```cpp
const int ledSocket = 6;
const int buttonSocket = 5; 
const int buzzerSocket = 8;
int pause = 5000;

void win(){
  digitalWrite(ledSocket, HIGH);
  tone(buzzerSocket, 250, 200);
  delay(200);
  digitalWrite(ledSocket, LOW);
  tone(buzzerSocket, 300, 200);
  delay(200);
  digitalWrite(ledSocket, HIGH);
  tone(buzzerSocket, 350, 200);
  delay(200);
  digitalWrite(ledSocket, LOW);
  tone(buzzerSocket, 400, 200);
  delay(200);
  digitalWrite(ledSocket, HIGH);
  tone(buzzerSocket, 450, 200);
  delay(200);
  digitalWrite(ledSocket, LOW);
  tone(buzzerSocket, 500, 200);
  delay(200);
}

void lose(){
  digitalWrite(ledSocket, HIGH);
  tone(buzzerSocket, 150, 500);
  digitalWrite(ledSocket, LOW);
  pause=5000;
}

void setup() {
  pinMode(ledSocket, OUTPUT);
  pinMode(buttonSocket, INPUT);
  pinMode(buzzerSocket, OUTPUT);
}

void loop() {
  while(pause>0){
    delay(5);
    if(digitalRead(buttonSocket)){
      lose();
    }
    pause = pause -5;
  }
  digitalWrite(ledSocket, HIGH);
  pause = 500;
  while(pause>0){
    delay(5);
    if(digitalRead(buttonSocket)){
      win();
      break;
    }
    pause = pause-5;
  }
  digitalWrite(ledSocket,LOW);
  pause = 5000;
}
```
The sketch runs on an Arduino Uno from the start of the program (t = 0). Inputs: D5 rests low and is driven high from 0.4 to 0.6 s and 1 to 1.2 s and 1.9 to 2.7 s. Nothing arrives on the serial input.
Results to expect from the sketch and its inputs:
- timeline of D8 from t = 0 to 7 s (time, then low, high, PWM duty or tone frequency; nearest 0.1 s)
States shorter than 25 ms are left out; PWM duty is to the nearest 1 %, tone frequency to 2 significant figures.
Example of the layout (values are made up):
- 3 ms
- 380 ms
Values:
- 0 s low; 0.4 s tone 150 Hz; 1.7 s low; 1.9 s tone 150 Hz; 3.2 s low
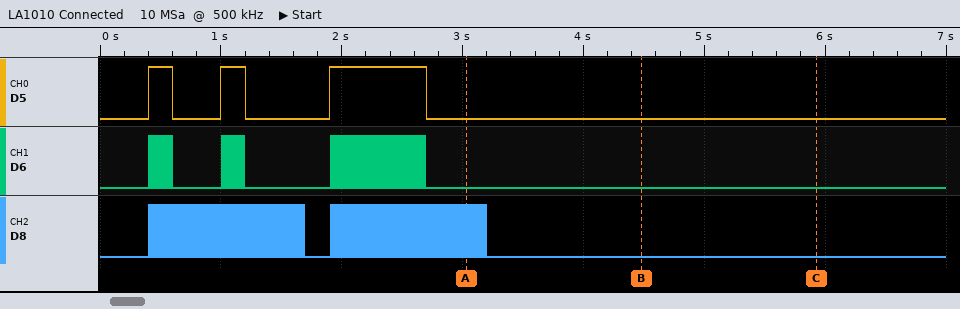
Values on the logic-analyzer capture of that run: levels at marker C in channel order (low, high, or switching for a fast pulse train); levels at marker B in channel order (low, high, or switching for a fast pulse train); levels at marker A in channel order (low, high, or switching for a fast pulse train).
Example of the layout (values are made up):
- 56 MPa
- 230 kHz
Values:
- D5 low, D6 low, D8 low
- D5 low, D6 low, D8 low
- D5 low, D6 low, D8 switching
